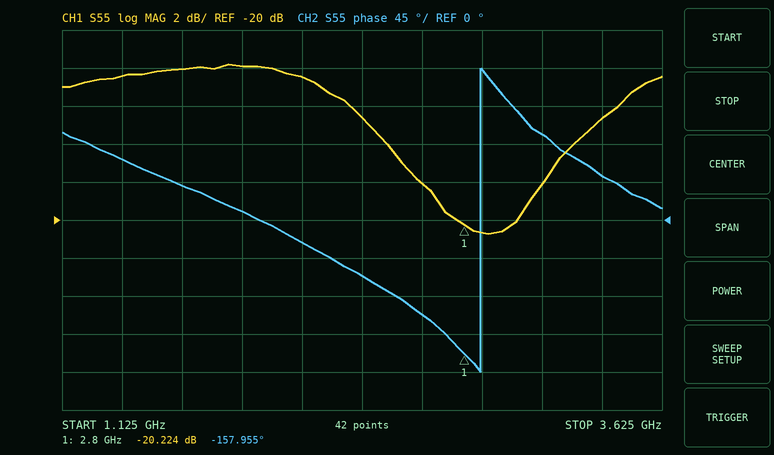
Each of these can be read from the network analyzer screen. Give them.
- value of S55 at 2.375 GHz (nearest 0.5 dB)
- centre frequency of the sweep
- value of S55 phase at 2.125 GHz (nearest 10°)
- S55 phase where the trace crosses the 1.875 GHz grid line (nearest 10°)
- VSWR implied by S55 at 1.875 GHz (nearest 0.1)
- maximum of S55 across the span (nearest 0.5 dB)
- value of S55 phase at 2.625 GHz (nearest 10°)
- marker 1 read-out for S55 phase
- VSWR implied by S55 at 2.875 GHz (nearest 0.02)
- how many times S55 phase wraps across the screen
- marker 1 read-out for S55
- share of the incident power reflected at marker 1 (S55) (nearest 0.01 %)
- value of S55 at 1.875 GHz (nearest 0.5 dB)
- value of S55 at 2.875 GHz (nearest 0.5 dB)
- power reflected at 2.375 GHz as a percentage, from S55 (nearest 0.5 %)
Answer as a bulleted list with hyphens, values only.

- -14.5 dB
- 2.375 GHz
- -30°
- 10°
- 1.7
- -12.0 dB
- -110°
- -157.955°
- 1.20
- 1
- -20.224 dB
- 0.95 %
- -12.0 dB
- -20.5 dB
- 3.5 %
